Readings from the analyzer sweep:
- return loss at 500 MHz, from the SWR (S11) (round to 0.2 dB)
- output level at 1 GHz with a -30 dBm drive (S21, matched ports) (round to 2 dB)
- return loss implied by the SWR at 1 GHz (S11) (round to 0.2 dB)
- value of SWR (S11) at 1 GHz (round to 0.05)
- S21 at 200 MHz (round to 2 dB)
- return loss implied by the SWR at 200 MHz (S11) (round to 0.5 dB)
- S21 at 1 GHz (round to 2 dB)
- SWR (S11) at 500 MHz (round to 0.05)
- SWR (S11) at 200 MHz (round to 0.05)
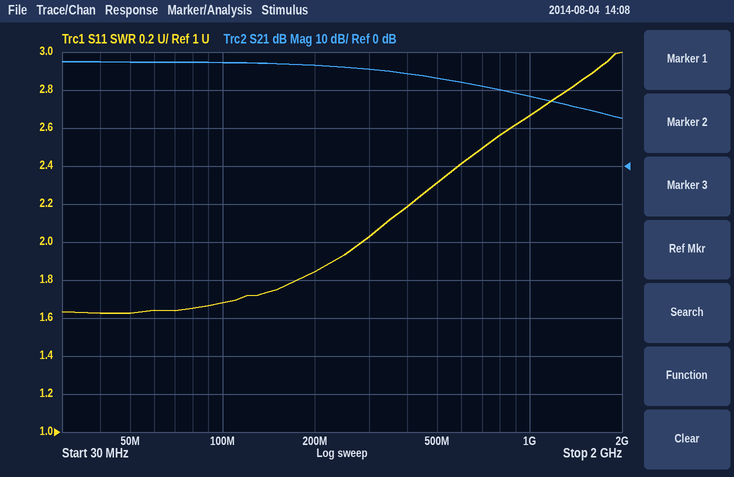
8.0 dB
-12 dBm
6.8 dB
2.65
26 dB
10.5 dB
18 dB
2.30
1.85
